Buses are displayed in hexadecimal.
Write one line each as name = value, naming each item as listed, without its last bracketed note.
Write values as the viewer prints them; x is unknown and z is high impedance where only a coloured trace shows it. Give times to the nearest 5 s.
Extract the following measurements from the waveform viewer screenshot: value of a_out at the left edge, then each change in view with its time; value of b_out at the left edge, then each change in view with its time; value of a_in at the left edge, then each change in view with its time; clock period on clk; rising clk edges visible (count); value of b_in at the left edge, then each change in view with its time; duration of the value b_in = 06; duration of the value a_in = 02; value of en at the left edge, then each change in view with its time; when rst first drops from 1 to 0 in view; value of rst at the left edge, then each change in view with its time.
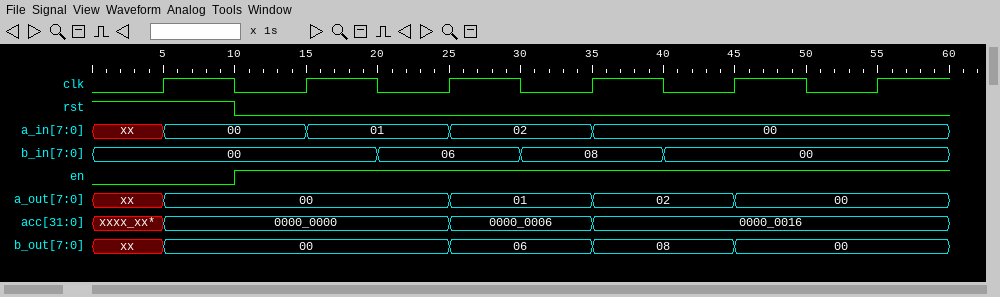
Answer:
value of a_out at the left edge, then each change in view with its time = xx, 00 at 5 s, 01 at 25 s, 02 at 35 s, 00 at 45 s
value of b_out at the left edge, then each change in view with its time = xx, 00 at 5 s, 06 at 25 s, 08 at 35 s, 00 at 45 s
value of a_in at the left edge, then each change in view with its time = xx, 00 at 5 s, 01 at 15 s, 02 at 25 s, 00 at 35 s
clock period on clk = 10 s
rising clk edges visible = 6
value of b_in at the left edge, then each change in view with its time = 00, 06 at 20 s, 08 at 30 s, 00 at 40 s
duration of the value b_in = 06 = 10 s
duration of the value a_in = 02 = 10 s
value of en at the left edge, then each change in view with its time = 0, 1 at 10 s
when rst first drops from 1 to 0 in view = 10 s
value of rst at the left edge, then each change in view with its time = 1, 0 at 10 s
